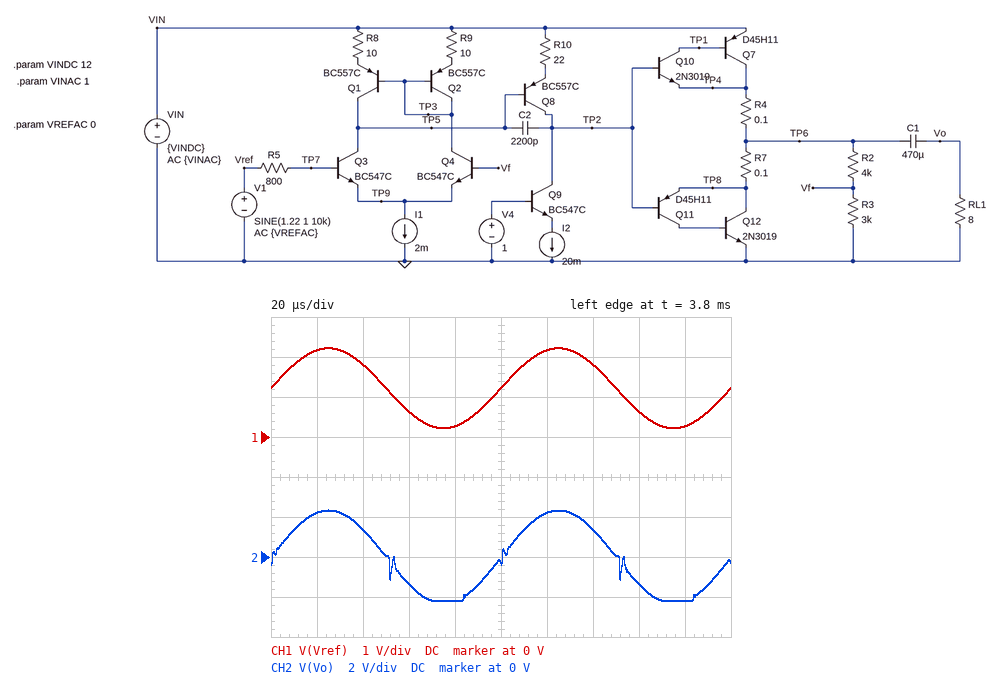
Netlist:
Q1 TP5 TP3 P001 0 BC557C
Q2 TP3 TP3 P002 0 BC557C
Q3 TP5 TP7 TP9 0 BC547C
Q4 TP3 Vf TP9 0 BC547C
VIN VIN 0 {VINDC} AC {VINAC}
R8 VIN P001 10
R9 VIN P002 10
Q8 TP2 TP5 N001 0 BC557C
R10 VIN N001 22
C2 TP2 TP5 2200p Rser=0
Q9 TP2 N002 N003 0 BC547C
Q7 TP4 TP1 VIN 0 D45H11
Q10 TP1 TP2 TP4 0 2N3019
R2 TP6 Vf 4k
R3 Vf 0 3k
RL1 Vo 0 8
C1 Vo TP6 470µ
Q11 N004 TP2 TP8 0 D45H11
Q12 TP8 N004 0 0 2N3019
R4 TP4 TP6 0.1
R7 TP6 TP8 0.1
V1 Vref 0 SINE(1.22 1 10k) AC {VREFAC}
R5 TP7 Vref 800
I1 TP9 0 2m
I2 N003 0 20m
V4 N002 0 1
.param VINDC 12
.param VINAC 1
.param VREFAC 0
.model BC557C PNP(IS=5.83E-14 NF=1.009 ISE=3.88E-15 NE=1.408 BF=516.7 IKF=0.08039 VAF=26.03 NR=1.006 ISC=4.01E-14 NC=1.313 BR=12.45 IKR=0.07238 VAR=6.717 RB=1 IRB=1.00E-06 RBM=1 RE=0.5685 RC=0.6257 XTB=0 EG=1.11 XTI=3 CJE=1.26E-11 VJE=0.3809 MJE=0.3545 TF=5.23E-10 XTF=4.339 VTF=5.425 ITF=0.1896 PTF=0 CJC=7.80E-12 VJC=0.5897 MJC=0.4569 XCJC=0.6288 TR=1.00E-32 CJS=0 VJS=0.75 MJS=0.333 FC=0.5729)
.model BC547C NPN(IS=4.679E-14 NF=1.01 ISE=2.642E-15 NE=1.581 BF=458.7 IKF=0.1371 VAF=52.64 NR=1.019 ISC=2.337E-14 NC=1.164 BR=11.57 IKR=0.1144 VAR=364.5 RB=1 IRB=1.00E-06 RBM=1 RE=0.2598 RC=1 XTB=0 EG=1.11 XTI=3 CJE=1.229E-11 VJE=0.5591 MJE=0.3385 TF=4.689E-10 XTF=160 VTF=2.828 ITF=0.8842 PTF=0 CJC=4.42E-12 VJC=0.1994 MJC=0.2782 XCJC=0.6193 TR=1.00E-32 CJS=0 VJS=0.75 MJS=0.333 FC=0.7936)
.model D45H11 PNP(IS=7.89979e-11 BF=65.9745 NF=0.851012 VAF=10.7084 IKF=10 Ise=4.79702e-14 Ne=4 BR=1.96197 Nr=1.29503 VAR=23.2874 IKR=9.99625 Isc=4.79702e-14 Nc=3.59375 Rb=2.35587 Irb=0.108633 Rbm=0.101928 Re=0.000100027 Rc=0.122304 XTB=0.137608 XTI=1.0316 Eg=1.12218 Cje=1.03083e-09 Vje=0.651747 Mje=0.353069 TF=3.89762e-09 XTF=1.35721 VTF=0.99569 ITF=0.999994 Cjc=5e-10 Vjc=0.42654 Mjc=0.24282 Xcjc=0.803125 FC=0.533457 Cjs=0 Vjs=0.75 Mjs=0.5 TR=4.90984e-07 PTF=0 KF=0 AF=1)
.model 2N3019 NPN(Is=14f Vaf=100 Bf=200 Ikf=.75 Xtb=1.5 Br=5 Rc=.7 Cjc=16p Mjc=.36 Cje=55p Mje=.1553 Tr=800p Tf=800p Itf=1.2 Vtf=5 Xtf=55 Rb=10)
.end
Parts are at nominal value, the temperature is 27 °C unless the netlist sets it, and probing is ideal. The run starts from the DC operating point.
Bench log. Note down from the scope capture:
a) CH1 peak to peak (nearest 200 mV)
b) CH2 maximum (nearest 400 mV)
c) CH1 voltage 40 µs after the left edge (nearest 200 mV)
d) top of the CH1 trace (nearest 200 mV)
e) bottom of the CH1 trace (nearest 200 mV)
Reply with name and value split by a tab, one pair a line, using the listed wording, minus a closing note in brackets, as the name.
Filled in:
CH1 peak to peak	2.0 V
CH2 maximum	2.4 V
CH1 voltage 40 µs after the left edge	1.8 V
top of the CH1 trace	2.2 V
bottom of the CH1 trace	200 mV
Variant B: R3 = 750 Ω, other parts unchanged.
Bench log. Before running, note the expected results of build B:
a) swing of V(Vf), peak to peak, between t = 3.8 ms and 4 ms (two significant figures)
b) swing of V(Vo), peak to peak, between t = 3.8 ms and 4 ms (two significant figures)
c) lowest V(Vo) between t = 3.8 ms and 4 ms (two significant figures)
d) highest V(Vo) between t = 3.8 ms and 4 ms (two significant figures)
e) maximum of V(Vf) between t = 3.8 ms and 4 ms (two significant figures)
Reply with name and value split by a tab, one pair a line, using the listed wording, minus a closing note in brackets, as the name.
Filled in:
swing of V(Vf), peak to peak, between t = 3.8 ms and 4 ms	1.5 V
swing of V(Vo), peak to peak, between t = 3.8 ms and 4 ms	9.4 V
lowest V(Vo) between t = 3.8 ms and 4 ms	-5.9 V
highest V(Vo) between t = 3.8 ms and 4 ms	3.5 V
maximum of V(Vf) between t = 3.8 ms and 4 ms	1.7 V
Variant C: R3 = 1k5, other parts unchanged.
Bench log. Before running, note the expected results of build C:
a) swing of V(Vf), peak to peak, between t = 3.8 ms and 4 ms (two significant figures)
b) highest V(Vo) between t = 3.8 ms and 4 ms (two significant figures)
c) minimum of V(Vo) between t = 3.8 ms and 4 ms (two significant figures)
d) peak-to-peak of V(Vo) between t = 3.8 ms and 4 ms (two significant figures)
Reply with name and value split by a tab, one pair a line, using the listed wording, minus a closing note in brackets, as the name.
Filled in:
swing of V(Vf), peak to peak, between t = 3.8 ms and 4 ms	2.0 V
highest V(Vo) between t = 3.8 ms and 4 ms	3.7 V
minimum of V(Vo) between t = 3.8 ms and 4 ms	-3.7 V
peak-to-peak of V(Vo) between t = 3.8 ms and 4 ms	7.3 V
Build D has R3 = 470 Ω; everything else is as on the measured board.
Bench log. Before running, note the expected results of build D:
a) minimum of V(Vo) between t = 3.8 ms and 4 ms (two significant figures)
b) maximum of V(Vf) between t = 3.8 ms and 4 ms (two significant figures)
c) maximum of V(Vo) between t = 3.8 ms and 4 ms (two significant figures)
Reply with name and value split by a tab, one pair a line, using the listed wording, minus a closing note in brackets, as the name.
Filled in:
minimum of V(Vo) between t = 3.8 ms and 4 ms	-7.1 V
maximum of V(Vf) between t = 3.8 ms and 4 ms	1.1 V
maximum of V(Vo) between t = 3.8 ms and 4 ms	1.7 V
